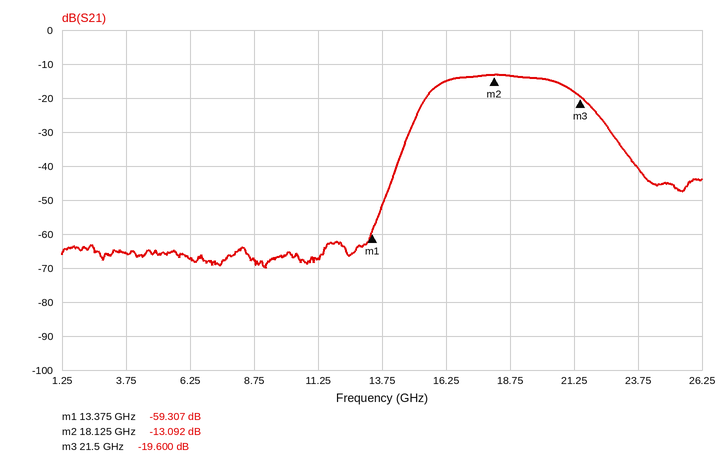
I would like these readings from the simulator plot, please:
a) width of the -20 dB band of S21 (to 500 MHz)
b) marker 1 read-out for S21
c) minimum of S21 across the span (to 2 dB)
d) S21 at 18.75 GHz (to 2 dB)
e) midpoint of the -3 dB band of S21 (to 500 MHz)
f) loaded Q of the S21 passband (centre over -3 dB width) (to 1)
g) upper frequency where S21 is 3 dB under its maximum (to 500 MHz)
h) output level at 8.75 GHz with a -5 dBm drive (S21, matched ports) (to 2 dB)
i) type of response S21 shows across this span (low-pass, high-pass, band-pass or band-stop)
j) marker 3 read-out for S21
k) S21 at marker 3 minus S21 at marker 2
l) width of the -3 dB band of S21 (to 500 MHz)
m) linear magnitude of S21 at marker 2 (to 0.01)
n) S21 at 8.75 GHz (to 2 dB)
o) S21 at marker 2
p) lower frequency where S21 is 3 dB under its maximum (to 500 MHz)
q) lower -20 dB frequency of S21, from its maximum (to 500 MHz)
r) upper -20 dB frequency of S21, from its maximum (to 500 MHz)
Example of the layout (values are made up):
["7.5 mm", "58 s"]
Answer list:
["8.5 GHz", "-59.307 dB", "-70 dB", "-14 dB", "18.5 GHz", "4", "21.0 GHz", "-72 dBm", "band-pass", "-19.600 dB", "-6.508 dB", "5.0 GHz", "0.22", "-68 dB", "-13.092 dB", "16.0 GHz", "14.5 GHz", "23.0 GHz"]
